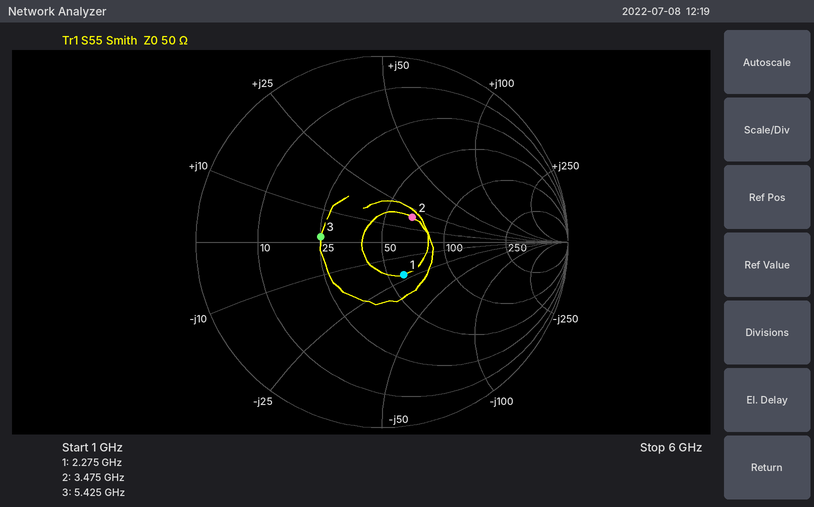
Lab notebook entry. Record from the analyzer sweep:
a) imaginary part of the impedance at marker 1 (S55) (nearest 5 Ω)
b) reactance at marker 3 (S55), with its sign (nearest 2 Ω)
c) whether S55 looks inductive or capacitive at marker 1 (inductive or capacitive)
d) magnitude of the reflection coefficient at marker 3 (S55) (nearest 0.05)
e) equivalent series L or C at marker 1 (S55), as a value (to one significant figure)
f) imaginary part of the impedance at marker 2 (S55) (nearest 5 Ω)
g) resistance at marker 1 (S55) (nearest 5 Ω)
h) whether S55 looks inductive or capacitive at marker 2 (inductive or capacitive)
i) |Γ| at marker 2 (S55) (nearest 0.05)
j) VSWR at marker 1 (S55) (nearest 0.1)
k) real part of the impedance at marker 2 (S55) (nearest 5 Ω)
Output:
-20 Ω
+2 Ω
capacitive
0.35
3 pF
+20 Ω
60 Ω
inductive
0.20
1.5
65 Ω
